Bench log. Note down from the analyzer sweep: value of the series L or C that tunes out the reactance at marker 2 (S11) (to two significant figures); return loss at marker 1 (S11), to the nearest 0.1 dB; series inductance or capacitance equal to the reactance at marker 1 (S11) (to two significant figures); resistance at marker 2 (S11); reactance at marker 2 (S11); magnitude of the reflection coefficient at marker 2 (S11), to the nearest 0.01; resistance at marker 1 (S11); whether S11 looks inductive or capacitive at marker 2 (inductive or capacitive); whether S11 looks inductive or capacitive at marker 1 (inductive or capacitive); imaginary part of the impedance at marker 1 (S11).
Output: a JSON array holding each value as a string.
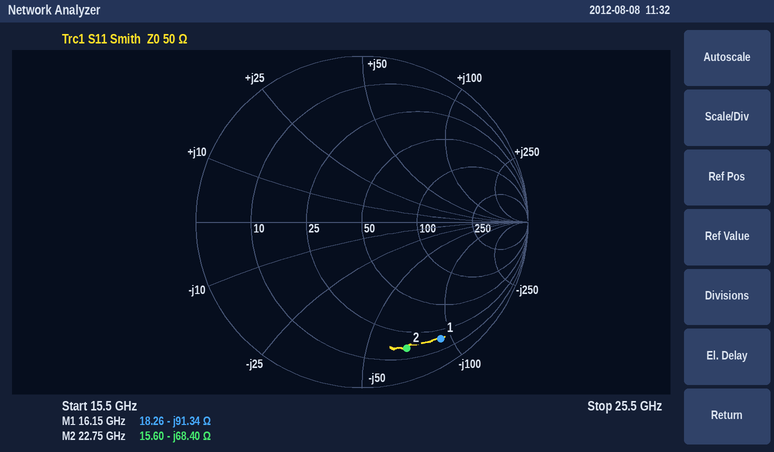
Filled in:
["480 pH", "1.4 dB", "110 fF", "15.60 Ω", "-68.40 Ω", "0.81", "18.26 Ω", "capacitive", "capacitive", "-91.34 Ω"]
